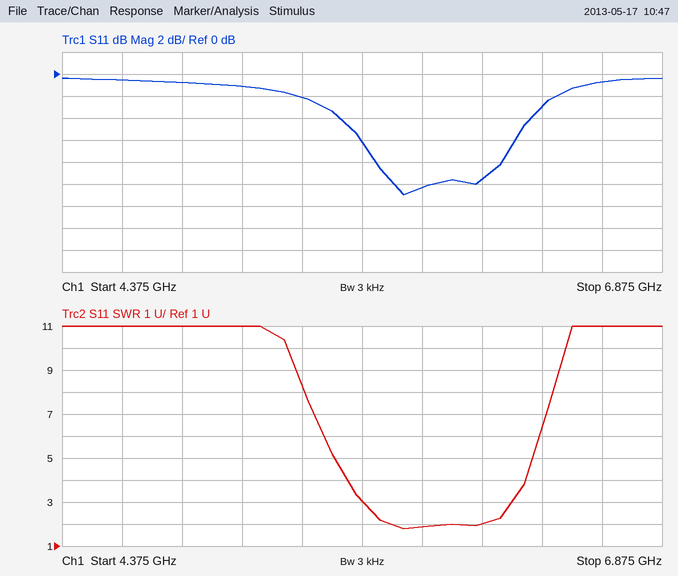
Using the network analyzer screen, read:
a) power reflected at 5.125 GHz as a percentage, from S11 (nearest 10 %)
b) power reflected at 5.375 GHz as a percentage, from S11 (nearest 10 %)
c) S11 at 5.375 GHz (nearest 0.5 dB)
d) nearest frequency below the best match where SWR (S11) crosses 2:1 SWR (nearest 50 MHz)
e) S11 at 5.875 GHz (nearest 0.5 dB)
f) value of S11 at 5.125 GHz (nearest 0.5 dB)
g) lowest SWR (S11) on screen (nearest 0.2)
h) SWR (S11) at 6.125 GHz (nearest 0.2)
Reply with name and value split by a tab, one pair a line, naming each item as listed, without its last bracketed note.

power reflected at 5.125 GHz as a percentage, from S11	80 %
power reflected at 5.375 GHz as a percentage, from S11	60 %
S11 at 5.375 GHz	-2.0 dB
nearest frequency below the best match where SWR (S11) crosses 2:1 SWR	5.75 GHz
S11 at 5.875 GHz	-10.5 dB
value of S11 at 5.125 GHz	-1.0 dB
lowest SWR (S11) on screen	1.8
SWR (S11) at 6.125 GHz	2.0
